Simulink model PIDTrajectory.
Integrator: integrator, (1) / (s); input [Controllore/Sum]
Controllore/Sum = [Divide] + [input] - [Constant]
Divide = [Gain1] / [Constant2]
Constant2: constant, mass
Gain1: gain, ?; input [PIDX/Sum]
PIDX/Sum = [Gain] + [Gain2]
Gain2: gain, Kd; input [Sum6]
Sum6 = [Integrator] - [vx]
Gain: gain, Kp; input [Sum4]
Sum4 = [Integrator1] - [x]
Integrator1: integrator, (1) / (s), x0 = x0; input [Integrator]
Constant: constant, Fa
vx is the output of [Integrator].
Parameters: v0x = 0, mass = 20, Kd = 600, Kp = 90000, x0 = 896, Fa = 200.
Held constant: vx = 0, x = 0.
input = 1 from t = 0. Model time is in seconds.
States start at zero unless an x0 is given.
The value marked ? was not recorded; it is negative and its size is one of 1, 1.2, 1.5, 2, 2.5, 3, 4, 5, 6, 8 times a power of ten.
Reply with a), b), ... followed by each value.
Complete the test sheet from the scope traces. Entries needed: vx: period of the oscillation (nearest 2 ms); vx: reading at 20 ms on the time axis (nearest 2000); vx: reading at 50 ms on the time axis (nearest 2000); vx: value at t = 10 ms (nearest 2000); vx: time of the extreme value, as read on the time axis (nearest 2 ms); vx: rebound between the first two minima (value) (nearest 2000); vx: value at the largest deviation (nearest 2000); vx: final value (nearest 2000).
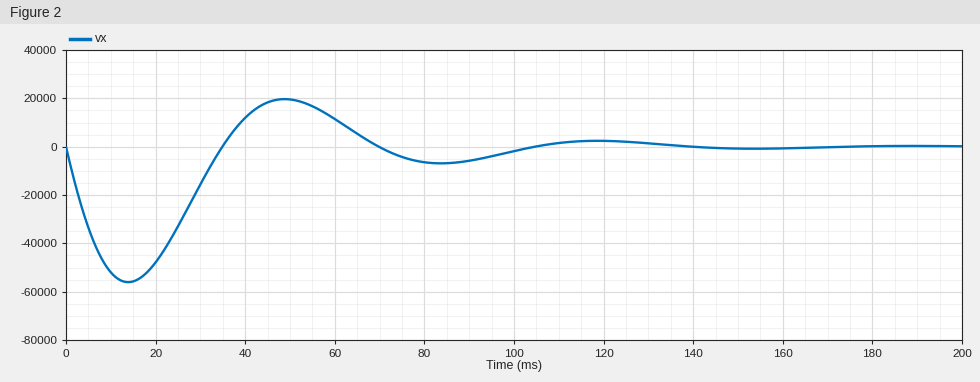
a) 70 ms
b) -48000
c) 20000
d) -52000
e) 14 ms
f) 20000
g) -56000
h) 0
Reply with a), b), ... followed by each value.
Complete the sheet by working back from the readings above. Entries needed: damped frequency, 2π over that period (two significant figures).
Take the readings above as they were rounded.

a) 0.090 rad/ms
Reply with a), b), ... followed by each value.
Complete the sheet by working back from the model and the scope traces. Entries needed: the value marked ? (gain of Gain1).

a) -2
